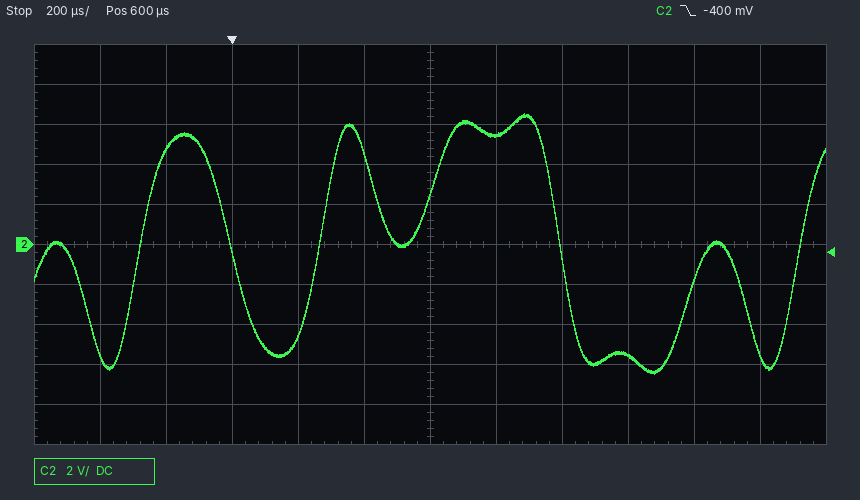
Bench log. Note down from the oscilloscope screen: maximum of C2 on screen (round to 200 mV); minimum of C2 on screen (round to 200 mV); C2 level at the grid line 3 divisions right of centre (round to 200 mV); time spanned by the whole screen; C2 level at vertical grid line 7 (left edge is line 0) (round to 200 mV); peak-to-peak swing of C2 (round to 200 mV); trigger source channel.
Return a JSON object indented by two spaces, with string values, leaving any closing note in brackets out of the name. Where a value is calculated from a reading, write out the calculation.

{
  "maximum of C2 on screen": "6.6 V",
  "minimum of C2 on screen": "-6.4 V",
  "C2 level at the grid line 3 divisions right of centre": "-5.6 V",
  "time spanned by the whole screen": "2.4 ms",
  "C2 level at vertical grid line 7 (left edge is line 0)": "5.4 V",
  "peak-to-peak swing of C2": "6.6 V − (-6.4 V) = 13.0 V",
  "trigger source channel": "C2"
}
